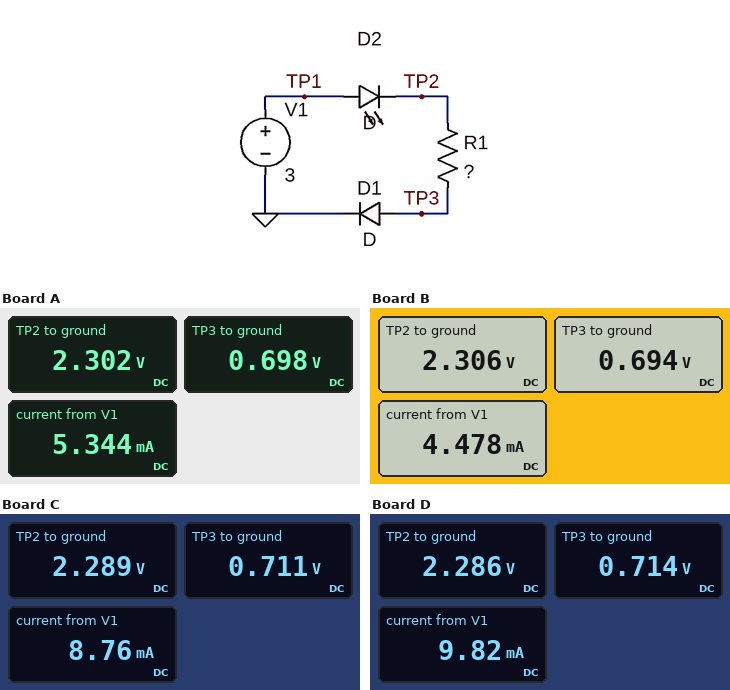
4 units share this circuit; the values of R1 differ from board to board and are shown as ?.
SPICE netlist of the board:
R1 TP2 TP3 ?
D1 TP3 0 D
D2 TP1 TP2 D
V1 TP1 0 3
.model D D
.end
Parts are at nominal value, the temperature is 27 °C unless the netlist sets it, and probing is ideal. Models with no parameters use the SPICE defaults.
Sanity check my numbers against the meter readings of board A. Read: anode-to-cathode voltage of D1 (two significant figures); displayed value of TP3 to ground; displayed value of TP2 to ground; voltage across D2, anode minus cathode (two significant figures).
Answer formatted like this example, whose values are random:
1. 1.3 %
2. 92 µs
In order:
1. 700 mV
2. 0.698 V
3. 2.302 V
4. 700 mV
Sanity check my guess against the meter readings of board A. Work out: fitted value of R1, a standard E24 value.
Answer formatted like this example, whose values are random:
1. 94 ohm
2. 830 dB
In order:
1. 300 Ω
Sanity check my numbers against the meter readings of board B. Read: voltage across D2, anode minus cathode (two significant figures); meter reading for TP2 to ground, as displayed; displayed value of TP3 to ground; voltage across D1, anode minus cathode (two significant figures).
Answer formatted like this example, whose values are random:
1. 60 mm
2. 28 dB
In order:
1. 690 mV
2. 2.306 V
3. 0.694 V
4. 690 mV
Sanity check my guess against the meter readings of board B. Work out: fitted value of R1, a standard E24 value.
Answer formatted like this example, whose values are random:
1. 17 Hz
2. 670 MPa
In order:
1. 360 Ω
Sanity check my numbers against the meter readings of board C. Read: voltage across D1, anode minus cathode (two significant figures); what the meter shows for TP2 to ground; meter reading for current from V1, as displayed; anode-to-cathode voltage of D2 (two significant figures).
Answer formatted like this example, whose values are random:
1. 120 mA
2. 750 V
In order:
1. 710 mV
2. 2.289 V
3. 8.76 mA
4. 710 mV
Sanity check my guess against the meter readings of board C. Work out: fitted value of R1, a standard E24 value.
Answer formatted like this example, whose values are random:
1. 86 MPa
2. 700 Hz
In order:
1. 180 Ω
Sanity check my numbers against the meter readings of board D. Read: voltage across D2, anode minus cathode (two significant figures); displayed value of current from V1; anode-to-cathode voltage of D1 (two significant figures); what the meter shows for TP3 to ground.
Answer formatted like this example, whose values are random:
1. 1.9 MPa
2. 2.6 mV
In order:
1. 710 mV
2. 9.82 mA
3. 710 mV
4. 0.714 V
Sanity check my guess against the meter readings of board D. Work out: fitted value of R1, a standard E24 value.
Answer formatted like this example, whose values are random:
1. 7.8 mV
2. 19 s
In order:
1. 160 Ω
